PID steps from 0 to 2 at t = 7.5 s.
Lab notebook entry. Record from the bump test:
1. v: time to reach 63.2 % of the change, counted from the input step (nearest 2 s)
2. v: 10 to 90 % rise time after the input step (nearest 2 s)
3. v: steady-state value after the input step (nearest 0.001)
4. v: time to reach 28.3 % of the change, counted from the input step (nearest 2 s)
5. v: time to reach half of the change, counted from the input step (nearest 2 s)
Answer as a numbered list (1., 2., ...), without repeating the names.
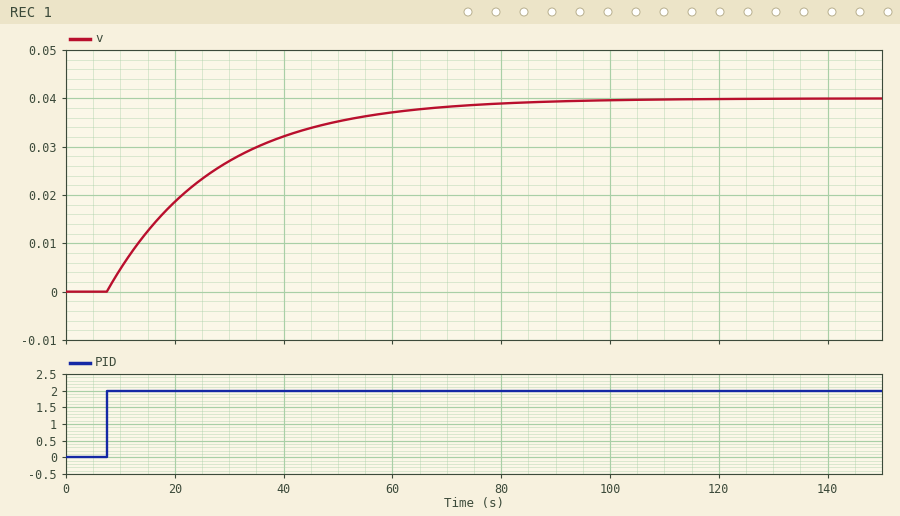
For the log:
1. 20 s
2. 44 s
3. 0.040
4. 6 s
5. 14 s
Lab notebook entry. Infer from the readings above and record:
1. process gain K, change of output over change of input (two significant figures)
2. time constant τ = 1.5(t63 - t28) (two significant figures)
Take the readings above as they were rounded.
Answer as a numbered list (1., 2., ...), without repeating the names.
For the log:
1. 0.020
2. 21 s
